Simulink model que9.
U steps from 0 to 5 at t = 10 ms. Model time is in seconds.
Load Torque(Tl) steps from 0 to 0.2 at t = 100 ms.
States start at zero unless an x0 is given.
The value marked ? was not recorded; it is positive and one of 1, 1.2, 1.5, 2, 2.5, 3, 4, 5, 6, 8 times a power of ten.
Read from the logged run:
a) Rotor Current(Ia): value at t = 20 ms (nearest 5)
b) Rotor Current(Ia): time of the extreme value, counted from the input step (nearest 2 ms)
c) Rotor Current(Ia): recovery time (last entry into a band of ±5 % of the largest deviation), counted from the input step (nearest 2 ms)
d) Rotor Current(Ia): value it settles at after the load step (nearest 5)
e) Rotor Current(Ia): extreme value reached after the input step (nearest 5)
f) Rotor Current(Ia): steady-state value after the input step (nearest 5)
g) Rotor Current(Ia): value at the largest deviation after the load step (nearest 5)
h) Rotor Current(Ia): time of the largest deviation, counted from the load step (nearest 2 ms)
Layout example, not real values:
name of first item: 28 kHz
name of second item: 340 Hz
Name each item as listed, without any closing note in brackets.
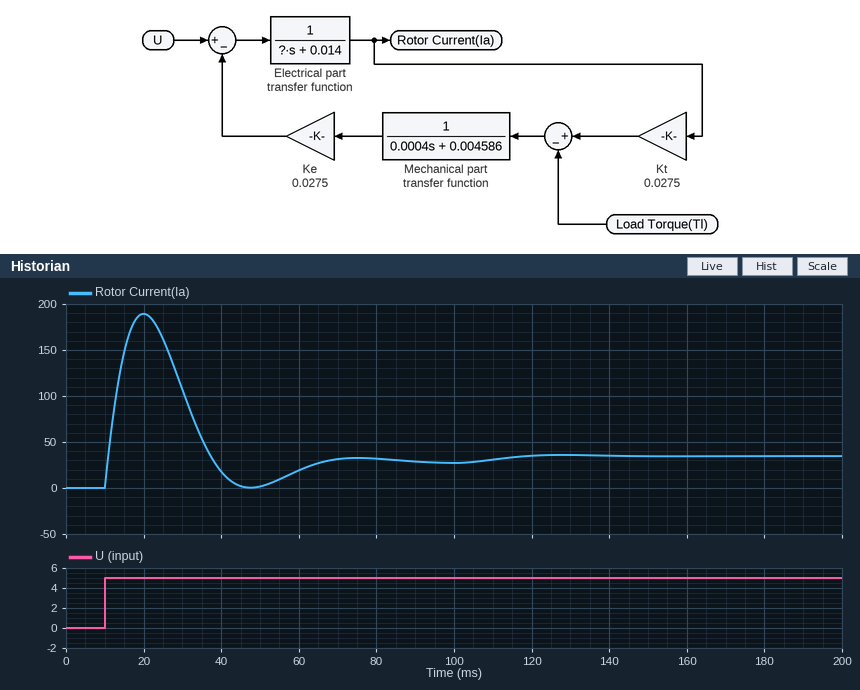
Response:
Rotor Current(Ia): value at t = 20 ms: 190
Rotor Current(Ia): time of the extreme value, counted from the input step: 10 ms
Rotor Current(Ia): recovery time (last entry into a band of ±5 % of the largest deviation), counted from the input step: 50 ms
Rotor Current(Ia): value it settles at after the load step: 35
Rotor Current(Ia): extreme value reached after the input step: 190
Rotor Current(Ia): steady-state value after the input step: 30
Rotor Current(Ia): value at the largest deviation after the load step: 35
Rotor Current(Ia): time of the largest deviation, counted from the load step: 28 ms
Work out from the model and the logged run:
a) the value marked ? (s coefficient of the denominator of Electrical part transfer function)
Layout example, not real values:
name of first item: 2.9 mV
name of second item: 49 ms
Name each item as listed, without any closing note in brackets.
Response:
the value marked ?: 0.00012
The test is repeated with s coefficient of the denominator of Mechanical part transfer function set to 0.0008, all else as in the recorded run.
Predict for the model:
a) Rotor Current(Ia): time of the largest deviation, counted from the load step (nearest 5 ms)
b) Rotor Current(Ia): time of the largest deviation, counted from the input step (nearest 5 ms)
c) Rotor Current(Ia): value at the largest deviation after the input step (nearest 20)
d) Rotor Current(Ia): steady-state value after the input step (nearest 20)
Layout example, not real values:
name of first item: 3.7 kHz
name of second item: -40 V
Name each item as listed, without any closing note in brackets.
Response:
Rotor Current(Ia): time of the largest deviation, counted from the load step: 40 ms
Rotor Current(Ia): time of the largest deviation, counted from the input step: 15 ms
Rotor Current(Ia): value at the largest deviation after the input step: 220
Rotor Current(Ia): steady-state value after the input step: 20
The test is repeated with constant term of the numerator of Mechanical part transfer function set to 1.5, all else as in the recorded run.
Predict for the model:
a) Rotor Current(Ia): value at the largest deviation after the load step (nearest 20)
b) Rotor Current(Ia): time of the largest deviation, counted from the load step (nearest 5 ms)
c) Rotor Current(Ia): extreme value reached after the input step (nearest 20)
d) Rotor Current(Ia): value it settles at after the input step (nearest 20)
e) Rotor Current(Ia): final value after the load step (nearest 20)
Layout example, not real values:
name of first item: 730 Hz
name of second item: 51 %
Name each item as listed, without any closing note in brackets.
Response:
Rotor Current(Ia): value at the largest deviation after the load step: 20
Rotor Current(Ia): time of the largest deviation, counted from the load step: 20 ms
Rotor Current(Ia): extreme value reached after the input step: 160
Rotor Current(Ia): value it settles at after the input step: 20
Rotor Current(Ia): final value after the load step: 20
